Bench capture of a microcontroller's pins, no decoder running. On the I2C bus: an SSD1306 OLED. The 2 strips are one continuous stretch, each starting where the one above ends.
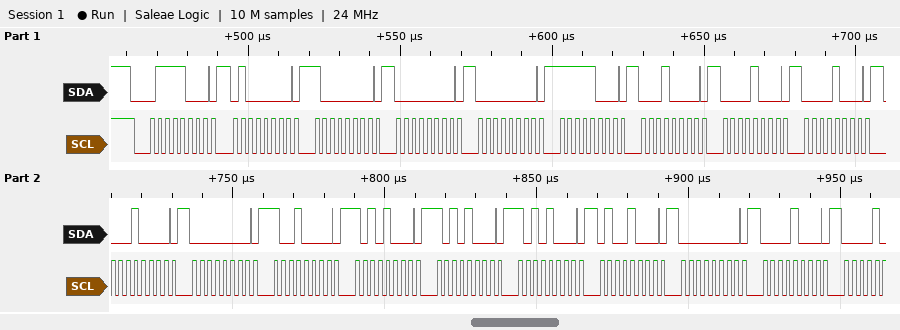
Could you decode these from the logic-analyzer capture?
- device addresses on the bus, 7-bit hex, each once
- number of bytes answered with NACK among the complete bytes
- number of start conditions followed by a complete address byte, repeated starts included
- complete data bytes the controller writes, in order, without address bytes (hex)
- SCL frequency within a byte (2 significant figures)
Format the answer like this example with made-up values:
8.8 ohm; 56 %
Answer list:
0x3C; 0; 1; 40 80 00 00 F8 10 08 08 10 00 90 A8 A8 A8 48 00 08; 400 kHz
